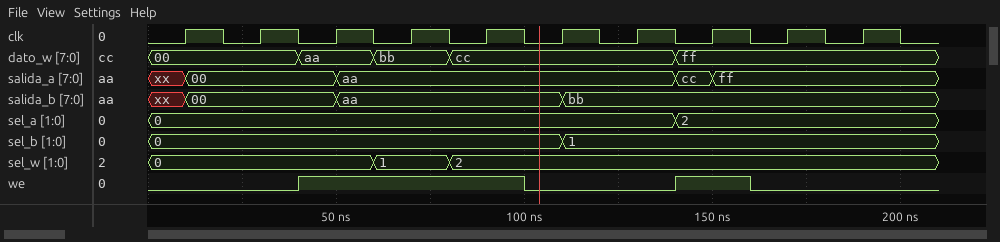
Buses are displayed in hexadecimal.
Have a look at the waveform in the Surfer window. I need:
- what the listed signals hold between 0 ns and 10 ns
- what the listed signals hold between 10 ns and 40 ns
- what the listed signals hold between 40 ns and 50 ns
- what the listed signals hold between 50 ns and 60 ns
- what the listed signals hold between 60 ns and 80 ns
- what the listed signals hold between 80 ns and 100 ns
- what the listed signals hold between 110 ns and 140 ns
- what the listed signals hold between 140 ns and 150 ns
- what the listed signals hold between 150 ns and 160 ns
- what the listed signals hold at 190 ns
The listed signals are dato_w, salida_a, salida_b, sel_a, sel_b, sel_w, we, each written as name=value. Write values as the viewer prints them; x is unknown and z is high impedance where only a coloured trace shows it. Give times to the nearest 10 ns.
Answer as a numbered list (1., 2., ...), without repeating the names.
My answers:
1. dato_w=00, salida_a=xx, salida_b=xx, sel_a=0, sel_b=0, sel_w=0, we=0
2. dato_w=00, salida_a=00, salida_b=00, sel_a=0, sel_b=0, sel_w=0, we=0
3. dato_w=aa, salida_a=00, salida_b=00, sel_a=0, sel_b=0, sel_w=0, we=1
4. dato_w=aa, salida_a=aa, salida_b=aa, sel_a=0, sel_b=0, sel_w=0, we=1
5. dato_w=bb, salida_a=aa, salida_b=aa, sel_a=0, sel_b=0, sel_w=1, we=1
6. dato_w=cc, salida_a=aa, salida_b=aa, sel_a=0, sel_b=0, sel_w=2, we=1
7. dato_w=cc, salida_a=aa, salida_b=bb, sel_a=0, sel_b=1, sel_w=2, we=0
8. dato_w=ff, salida_a=cc, salida_b=bb, sel_a=2, sel_b=1, sel_w=2, we=1
9. dato_w=ff, salida_a=ff, salida_b=bb, sel_a=2, sel_b=1, sel_w=2, we=1
10. dato_w=ff, salida_a=ff, salida_b=bb, sel_a=2, sel_b=1, sel_w=2, we=0
